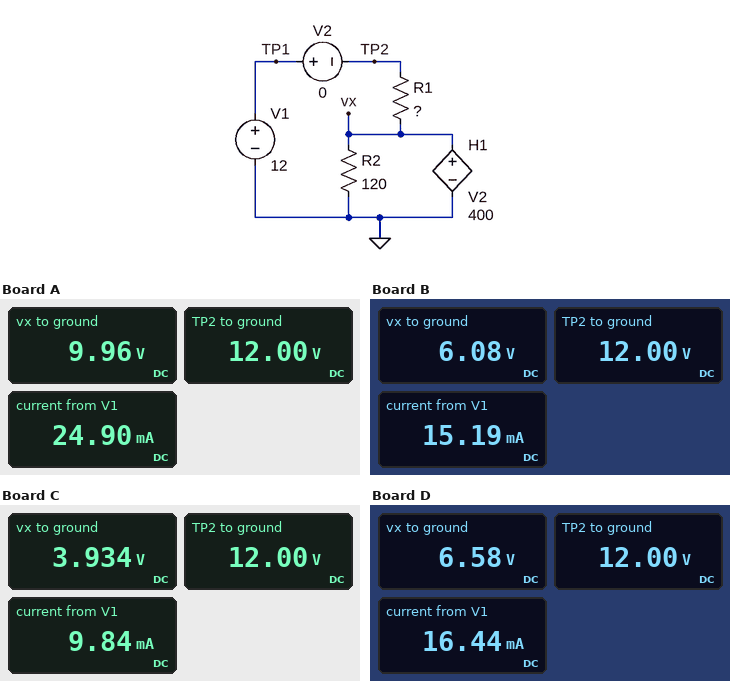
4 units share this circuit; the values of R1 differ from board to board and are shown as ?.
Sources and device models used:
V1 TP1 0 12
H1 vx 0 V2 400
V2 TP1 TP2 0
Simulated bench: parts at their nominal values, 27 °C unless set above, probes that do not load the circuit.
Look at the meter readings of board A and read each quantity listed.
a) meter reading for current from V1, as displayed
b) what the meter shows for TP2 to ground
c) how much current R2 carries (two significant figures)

24.90 mA
12.00 V
83 mA
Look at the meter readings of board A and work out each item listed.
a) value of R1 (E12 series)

82 Ω
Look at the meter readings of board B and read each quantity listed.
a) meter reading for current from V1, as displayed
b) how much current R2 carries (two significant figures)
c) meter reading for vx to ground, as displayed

15.19 mA
51 mA
6.08 V
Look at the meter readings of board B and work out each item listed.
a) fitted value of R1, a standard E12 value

390 Ω
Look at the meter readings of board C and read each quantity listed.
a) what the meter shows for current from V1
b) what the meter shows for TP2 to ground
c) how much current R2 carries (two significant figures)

9.84 mA
12.00 V
33 mA
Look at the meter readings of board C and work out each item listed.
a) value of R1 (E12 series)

820 Ω
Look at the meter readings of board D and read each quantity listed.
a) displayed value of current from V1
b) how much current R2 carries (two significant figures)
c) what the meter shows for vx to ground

16.44 mA
55 mA
6.58 V
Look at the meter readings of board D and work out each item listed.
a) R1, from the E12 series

330 Ω
